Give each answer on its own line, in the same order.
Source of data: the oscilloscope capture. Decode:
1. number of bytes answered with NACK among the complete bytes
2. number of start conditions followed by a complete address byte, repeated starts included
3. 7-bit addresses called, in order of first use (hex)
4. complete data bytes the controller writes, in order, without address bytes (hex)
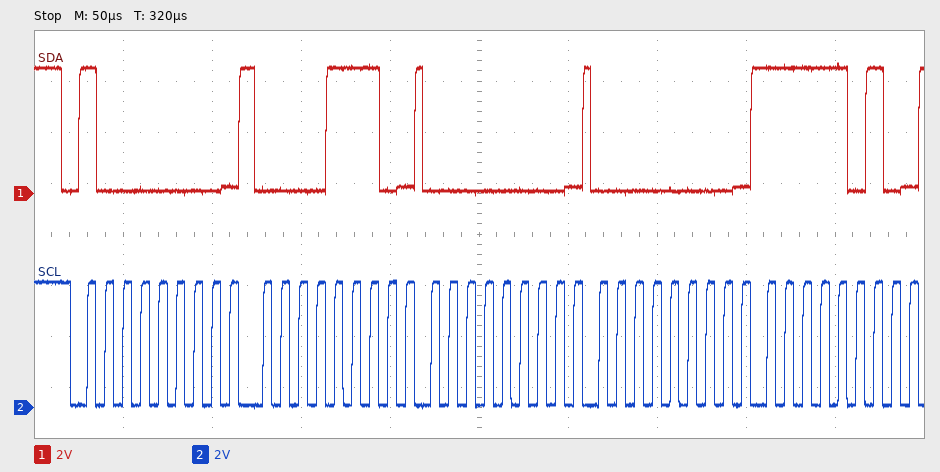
0
1
0x40
0E 00 00 FA
